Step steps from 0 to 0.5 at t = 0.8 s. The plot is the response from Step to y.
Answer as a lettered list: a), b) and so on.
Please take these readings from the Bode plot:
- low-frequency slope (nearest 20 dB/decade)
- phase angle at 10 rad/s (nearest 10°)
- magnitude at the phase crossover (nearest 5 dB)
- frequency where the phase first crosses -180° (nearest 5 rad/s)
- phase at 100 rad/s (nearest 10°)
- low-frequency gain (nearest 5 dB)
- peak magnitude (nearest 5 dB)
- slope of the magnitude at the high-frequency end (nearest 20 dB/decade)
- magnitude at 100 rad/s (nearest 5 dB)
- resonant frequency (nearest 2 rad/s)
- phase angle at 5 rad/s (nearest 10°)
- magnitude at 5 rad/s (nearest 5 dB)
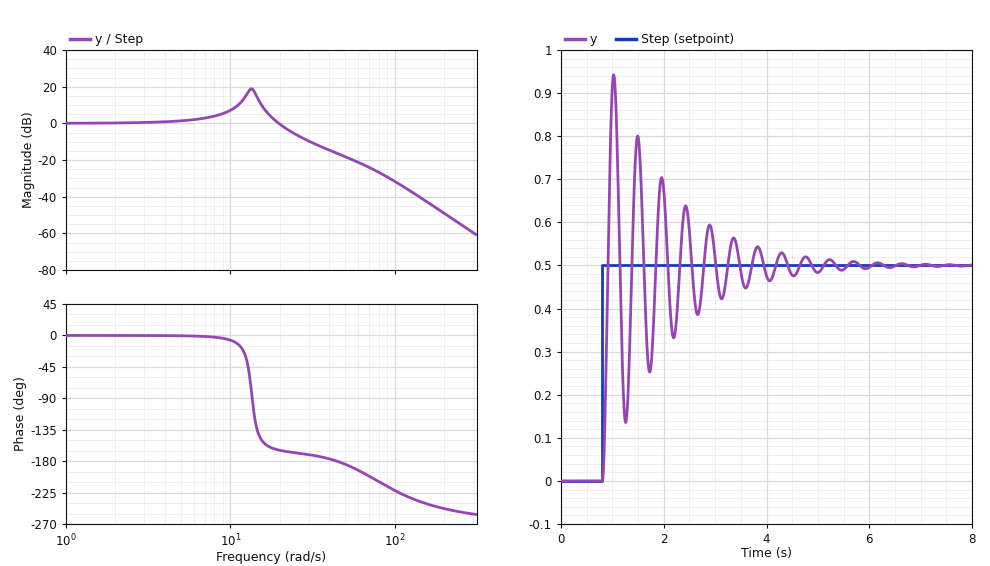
a) 0 dB/decade
b) -10°
c) -15 dB
d) 45 rad/s
e) -220°
f) 0 dB
g) 20 dB
h) -60 dB/decade
i) -30 dB
j) 14 rad/s
k) 0°
l) 0 dB
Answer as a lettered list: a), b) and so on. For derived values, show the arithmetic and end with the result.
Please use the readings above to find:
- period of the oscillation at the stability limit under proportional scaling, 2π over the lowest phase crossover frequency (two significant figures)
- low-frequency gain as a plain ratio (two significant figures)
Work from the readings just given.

a) 2π / 45 = 0.14 s
b) 10^(0 / 20) = 1.0
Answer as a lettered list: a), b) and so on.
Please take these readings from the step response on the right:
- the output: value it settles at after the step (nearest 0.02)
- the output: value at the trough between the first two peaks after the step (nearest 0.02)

a) 0.50
b) 0.14
